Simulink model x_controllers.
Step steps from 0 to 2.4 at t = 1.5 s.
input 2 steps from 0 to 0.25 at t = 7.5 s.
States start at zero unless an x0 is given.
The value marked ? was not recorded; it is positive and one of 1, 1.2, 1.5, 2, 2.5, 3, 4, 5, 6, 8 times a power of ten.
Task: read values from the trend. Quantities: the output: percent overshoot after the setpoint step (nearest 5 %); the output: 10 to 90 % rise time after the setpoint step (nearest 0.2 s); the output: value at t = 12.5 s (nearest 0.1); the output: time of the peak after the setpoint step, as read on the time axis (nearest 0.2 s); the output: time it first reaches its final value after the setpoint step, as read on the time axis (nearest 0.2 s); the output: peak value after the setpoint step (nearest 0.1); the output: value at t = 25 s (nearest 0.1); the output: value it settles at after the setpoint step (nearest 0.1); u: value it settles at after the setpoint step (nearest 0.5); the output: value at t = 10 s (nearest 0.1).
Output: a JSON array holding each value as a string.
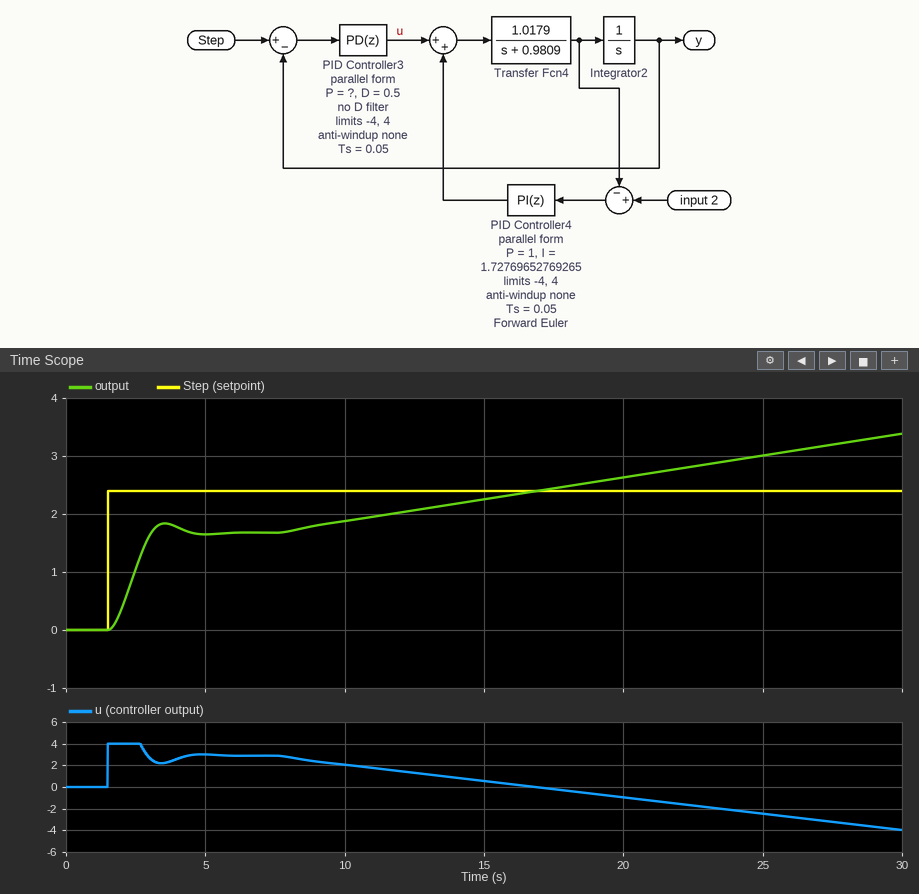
["10 %", "1.0 s", "2.1", "3.6 s", "3.0 s", "1.8", "3.0", "1.7", "3.0", "1.9"]
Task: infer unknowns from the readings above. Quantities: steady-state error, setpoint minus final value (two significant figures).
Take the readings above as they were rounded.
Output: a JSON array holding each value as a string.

["0.70"]
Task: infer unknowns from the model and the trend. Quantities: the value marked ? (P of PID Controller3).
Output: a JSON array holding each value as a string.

["4"]
